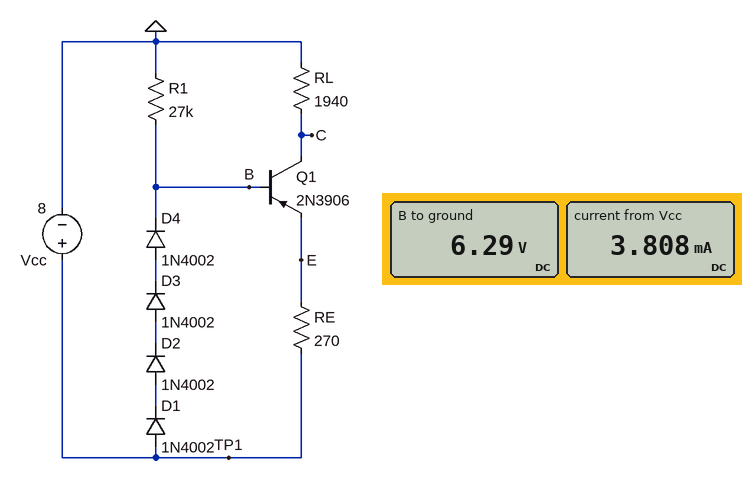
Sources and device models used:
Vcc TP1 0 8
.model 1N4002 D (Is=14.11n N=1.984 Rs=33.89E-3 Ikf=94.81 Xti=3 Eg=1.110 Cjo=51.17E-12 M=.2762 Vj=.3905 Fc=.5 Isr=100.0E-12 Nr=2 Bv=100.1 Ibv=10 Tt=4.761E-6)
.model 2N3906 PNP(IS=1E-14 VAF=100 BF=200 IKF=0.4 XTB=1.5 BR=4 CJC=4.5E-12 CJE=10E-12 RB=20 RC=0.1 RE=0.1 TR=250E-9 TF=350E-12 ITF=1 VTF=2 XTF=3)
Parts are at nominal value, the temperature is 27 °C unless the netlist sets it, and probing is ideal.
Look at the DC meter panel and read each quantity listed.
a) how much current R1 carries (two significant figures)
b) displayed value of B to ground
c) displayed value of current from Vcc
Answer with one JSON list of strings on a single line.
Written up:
["230 µA", "6.29 V", "3.808 mA"]
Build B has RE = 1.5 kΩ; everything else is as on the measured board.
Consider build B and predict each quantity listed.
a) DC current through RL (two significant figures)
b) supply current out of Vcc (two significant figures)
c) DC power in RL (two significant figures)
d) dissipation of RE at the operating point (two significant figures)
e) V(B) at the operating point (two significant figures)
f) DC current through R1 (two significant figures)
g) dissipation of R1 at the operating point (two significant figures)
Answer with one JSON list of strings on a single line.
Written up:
["880 µA", "1.1 mA", "1.5 mW", "1.2 mW", "6.0 V", "220 µA", "1.3 mW"]
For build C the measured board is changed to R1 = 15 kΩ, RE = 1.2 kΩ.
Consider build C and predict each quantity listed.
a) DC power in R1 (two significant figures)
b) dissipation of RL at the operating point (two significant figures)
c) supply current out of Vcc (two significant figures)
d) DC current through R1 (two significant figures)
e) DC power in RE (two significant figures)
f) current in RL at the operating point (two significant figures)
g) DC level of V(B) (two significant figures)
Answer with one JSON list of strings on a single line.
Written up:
["2.3 mW", "2.8 mW", "1.6 mA", "390 µA", "1.7 mW", "1.2 mA", "5.9 V"]
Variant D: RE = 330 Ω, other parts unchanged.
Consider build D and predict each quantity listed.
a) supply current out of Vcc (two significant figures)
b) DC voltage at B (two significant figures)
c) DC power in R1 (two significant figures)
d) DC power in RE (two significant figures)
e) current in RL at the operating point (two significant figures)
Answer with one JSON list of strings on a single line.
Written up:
["3.7 mA", "6.1 V", "1.4 mW", "4.2 mW", "3.5 mA"]
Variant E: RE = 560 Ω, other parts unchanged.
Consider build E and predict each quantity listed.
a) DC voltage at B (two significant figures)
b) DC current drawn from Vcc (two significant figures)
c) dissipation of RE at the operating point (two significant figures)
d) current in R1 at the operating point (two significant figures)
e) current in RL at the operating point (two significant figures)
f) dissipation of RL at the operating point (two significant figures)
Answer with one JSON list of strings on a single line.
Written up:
["6.0 V", "2.5 mA", "3.0 mW", "220 µA", "2.3 mA", "10 mW"]
